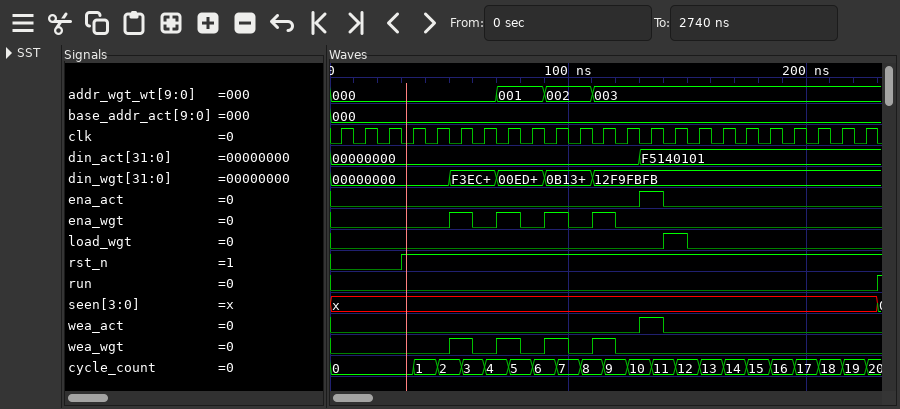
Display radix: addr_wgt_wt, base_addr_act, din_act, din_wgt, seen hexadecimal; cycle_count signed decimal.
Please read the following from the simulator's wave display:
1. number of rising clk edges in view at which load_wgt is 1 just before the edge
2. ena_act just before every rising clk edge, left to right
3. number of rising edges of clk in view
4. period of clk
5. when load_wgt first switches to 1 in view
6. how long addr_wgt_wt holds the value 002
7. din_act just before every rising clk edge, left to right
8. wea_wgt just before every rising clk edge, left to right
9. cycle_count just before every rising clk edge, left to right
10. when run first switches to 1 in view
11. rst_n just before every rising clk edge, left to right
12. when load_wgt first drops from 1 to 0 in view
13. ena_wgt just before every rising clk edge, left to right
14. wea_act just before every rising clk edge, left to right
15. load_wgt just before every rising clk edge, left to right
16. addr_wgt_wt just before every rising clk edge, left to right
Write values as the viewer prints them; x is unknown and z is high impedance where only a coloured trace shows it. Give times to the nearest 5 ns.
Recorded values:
1
0 0 0 0 0 0 0 0 0 0 0 0 0 1 0 0 0 0 0 0 0 0 0
23
10 ns
140 ns
20 ns
00000000, 00000000, 00000000, 00000000, 00000000, 00000000, 00000000, 00000000, 00000000, 00000000, 00000000, 00000000, 00000000, F5140101, F5140101, F5140101, F5140101, F5140101, F5140101, F5140101, F5140101, F5140101, F5140101
0 0 0 0 0 1 0 1 0 1 0 1 0 0 0 0 0 0 0 0 0 0 0
0, 0, 0, 0, 1, 2, 3, 4, 5, 6, 7, 8, 9, 10, 11, 12, 13, 14, 15, 16, 17, 18, 19
230 ns
0 0 0 1 1 1 1 1 1 1 1 1 1 1 1 1 1 1 1 1 1 1 1
150 ns
0 0 0 0 0 1 0 1 0 1 0 1 0 0 0 0 0 0 0 0 0 0 0
0 0 0 0 0 0 0 0 0 0 0 0 0 1 0 0 0 0 0 0 0 0 0
0 0 0 0 0 0 0 0 0 0 0 0 0 0 1 0 0 0 0 0 0 0 0
000, 000, 000, 000, 000, 000, 000, 001, 001, 002, 002, 003, 003, 003, 003, 003, 003, 003, 003, 003, 003, 003, 003
